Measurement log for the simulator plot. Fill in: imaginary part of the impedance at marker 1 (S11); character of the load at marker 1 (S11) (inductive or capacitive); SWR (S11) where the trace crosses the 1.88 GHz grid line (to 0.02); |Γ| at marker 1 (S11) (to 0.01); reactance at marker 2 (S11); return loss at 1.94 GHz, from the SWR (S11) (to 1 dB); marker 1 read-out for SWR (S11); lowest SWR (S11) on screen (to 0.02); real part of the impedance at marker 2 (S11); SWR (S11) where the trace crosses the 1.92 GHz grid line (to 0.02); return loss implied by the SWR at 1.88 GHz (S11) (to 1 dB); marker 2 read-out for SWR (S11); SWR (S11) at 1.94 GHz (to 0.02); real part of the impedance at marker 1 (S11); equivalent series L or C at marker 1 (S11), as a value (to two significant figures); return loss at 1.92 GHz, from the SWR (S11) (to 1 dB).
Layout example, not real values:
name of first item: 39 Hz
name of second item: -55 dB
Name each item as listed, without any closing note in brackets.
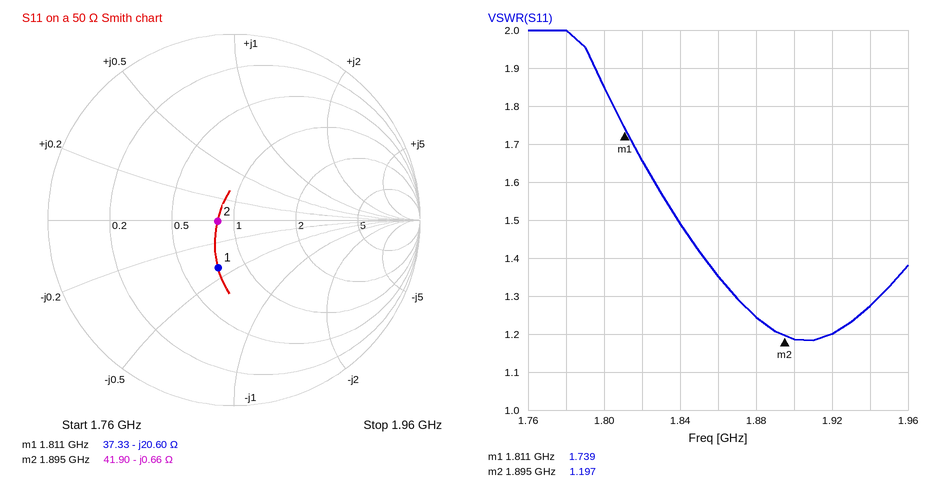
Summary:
imaginary part of the impedance at marker 1: -20.60 Ω
character of the load at marker 1 (S11): capacitive
SWR (S11) where the trace crosses the 1.88 GHz grid line: 1.24
|Γ| at marker 1 (S11): 0.27
reactance at marker 2: -0.66 Ω
return loss at 1.94 GHz, from the SWR (S11): 18 dB
marker 1 read-out for SWR: 1.739
lowest SWR (S11) on screen: 1.18
real part of the impedance at marker 2: 41.90 Ω
SWR (S11) where the trace crosses the 1.92 GHz grid line: 1.20
return loss implied by the SWR at 1.88 GHz (S11): 19 dB
marker 2 read-out for SWR: 1.197
SWR (S11) at 1.94 GHz: 1.28
real part of the impedance at marker 1: 37.33 Ω
equivalent series L or C at marker 1 (S11), as a value: 4.3 pF
return loss at 1.92 GHz, from the SWR (S11): 21 dB
